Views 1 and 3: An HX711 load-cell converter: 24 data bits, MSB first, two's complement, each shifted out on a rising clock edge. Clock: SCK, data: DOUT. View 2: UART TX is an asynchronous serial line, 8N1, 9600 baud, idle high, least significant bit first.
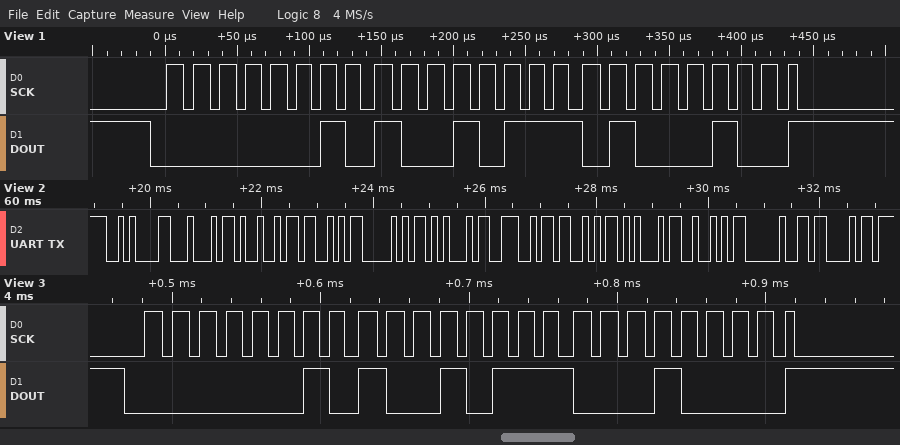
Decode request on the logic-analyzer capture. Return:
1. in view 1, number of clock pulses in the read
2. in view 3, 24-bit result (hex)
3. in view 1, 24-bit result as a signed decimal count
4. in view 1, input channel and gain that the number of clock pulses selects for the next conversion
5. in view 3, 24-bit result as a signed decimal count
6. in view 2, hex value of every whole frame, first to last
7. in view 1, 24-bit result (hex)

25
0x029710
169796
channel A, gain 128
169744
0A 44 49 53 50 45 4E 53 45 52 20 43
0x029744
